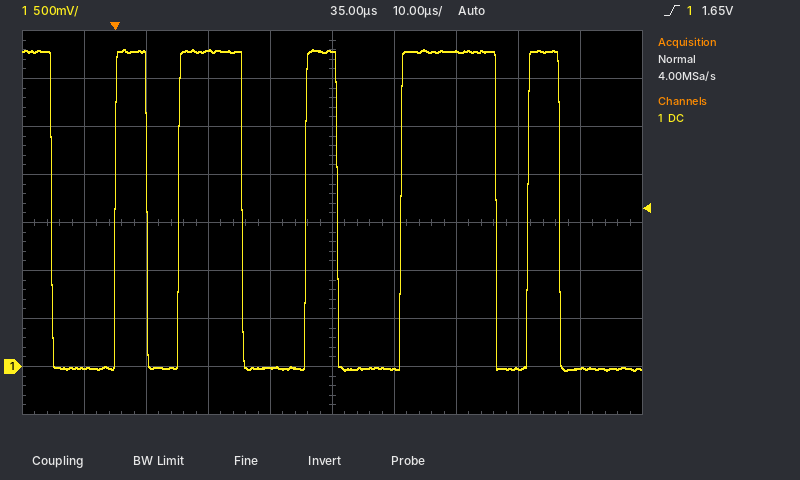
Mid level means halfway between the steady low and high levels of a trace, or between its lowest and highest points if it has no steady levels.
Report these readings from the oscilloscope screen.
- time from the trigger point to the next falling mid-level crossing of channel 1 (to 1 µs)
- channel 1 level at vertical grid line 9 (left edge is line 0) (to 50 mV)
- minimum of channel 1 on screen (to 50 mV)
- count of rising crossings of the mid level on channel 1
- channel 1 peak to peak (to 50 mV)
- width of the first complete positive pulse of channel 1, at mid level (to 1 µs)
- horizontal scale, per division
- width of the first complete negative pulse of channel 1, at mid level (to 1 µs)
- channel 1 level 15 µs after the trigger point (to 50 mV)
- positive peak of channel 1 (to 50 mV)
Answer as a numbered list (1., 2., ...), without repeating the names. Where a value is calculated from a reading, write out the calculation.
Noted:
1. 5 µs
2. 0 mV
3. -50 mV
4. 5
5. 3.30 V − (-50 mV) = 3.35 V
6. 5 µs
7. 10 µs
8. 10 µs
9. 3.30 V
10. 3.30 V
